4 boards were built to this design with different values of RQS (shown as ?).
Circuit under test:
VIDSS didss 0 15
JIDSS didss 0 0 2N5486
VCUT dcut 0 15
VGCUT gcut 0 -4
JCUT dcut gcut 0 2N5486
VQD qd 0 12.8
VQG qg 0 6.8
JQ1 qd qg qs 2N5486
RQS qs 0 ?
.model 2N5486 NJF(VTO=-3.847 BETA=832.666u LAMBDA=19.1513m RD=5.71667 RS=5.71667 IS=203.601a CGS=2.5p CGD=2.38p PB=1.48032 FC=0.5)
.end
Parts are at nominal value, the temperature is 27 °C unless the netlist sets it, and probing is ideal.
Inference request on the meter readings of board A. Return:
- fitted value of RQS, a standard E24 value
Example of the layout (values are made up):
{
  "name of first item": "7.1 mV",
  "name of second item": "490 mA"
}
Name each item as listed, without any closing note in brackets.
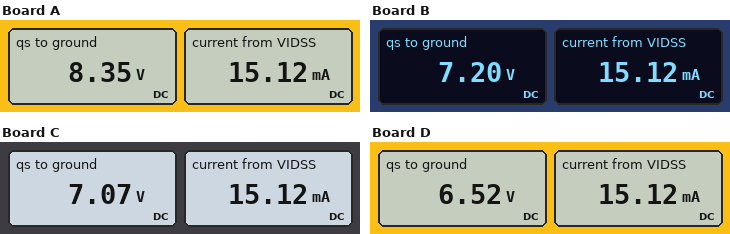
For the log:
{
  "fitted value of RQS, a standard E24 value": "1.8 kΩ"
}
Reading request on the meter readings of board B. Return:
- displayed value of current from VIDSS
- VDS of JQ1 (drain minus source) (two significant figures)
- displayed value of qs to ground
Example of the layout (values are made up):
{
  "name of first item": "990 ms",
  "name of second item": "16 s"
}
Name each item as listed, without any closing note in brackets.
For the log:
{
  "displayed value of current from VIDSS": "15.12 mA",
  "VDS of JQ1 (drain minus source)": "5.6 V",
  "displayed value of qs to ground": "7.20 V"
}
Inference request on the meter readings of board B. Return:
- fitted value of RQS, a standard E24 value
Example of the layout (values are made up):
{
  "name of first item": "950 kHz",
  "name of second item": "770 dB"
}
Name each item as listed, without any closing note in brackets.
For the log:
{
  "fitted value of RQS, a standard E24 value": "680 Ω"
}
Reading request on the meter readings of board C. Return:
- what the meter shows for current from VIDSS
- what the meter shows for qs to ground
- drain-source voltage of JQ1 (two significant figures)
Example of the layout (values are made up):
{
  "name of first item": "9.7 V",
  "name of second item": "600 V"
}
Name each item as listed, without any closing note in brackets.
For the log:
{
  "what the meter shows for current from VIDSS": "15.12 mA",
  "what the meter shows for qs to ground": "7.07 V",
  "drain-source voltage of JQ1": "5.7 V"
}
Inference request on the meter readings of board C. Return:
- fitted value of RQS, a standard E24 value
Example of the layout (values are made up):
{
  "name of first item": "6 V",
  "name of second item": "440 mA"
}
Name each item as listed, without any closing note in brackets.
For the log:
{
  "fitted value of RQS, a standard E24 value": "620 Ω"
}
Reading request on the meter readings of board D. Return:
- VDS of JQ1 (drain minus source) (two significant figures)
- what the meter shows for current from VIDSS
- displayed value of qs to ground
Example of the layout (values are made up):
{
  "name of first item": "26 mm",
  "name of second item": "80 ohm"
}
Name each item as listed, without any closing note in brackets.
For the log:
{
  "VDS of JQ1 (drain minus source)": "6.3 V",
  "what the meter shows for current from VIDSS": "15.12 mA",
  "displayed value of qs to ground": "6.52 V"
}
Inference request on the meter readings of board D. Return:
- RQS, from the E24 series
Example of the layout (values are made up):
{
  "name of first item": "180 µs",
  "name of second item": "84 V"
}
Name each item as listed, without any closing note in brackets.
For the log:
{
  "RQS, from the E24 series": "430 Ω"
}
